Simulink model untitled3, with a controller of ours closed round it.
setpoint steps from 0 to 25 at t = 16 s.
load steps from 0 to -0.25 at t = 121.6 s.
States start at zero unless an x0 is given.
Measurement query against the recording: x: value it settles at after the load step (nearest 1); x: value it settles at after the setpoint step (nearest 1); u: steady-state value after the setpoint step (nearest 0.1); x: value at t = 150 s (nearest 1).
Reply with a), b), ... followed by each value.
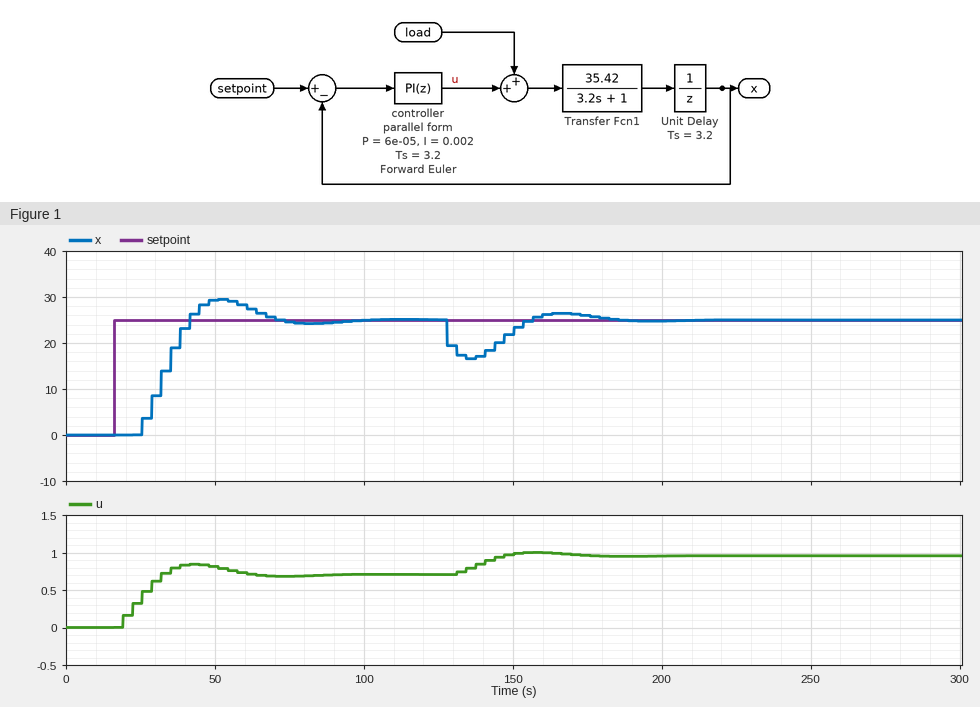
a) 25
b) 25
c) 0.7
d) 22
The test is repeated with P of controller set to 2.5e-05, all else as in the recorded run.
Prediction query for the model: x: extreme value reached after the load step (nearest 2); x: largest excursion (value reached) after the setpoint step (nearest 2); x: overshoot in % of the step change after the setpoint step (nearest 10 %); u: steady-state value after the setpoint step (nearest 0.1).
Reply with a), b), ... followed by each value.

a) 16
b) 30
c) 20 %
d) 0.7
